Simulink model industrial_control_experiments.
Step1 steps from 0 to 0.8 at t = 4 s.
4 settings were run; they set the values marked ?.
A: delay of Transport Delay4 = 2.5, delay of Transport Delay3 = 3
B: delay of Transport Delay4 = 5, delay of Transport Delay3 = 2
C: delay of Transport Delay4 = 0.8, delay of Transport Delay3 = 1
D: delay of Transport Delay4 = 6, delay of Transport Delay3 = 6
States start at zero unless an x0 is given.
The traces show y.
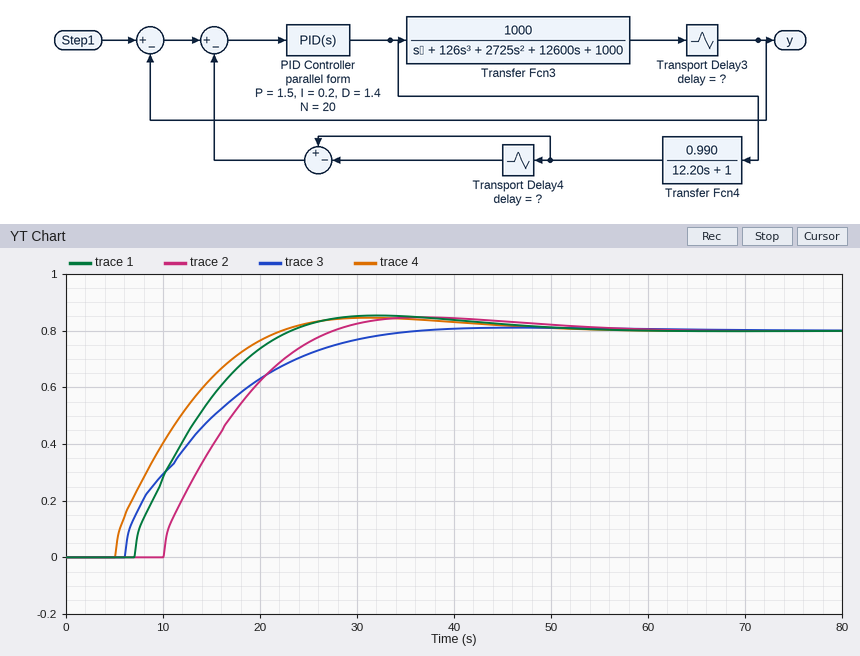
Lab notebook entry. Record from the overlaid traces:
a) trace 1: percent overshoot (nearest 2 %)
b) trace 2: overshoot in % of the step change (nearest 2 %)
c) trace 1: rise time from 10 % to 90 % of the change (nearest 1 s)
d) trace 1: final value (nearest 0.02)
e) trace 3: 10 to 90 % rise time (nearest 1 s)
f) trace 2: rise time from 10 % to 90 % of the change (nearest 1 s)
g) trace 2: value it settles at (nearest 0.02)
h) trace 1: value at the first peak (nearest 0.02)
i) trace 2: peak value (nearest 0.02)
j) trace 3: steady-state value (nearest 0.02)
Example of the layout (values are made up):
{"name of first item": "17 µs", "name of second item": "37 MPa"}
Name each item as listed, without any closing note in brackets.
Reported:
{"trace 1: percent overshoot": "6 %", "trace 2: overshoot in % of the step change": "6 %", "trace 1: rise time from 10 % to 90 % of the change": "12 s", "trace 1: final value": "0.80", "trace 3: 10 to 90 % rise time": "19 s", "trace 2: rise time from 10 % to 90 % of the change": "13 s", "trace 2: value it settles at": "0.80", "trace 1: value at the first peak": "0.86", "trace 2: peak value": "0.84", "trace 3: steady-state value": "0.80"}
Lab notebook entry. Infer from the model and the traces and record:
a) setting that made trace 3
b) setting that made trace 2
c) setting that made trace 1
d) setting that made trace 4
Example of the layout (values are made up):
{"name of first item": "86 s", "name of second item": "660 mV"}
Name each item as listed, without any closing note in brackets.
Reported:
{"setting that made trace 3": "B", "setting that made trace 2": "D", "setting that made trace 1": "A", "setting that made trace 4": "C"}
